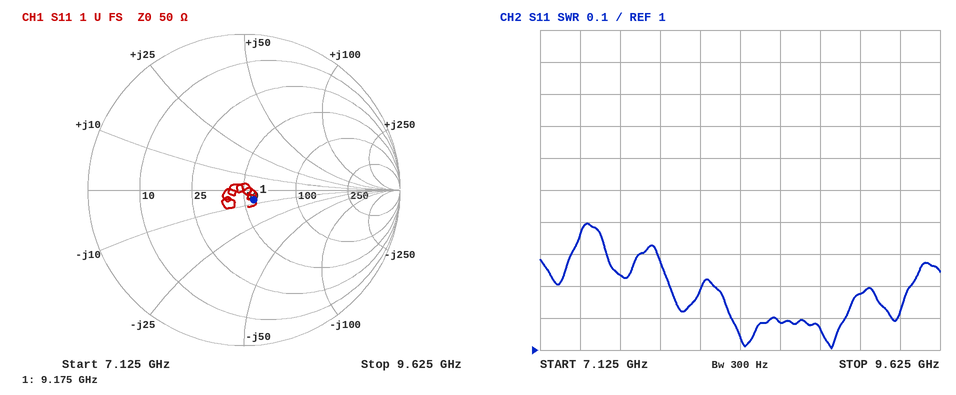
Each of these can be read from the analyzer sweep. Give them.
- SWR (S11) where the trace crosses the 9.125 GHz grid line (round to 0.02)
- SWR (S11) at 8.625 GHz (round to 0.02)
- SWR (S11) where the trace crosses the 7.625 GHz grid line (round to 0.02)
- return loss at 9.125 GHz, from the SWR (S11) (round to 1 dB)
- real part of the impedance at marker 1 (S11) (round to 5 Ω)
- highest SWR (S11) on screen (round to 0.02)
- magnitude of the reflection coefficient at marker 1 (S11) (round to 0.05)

1.18
1.08
1.24
22 dB
55 Ω
1.40
0.10
